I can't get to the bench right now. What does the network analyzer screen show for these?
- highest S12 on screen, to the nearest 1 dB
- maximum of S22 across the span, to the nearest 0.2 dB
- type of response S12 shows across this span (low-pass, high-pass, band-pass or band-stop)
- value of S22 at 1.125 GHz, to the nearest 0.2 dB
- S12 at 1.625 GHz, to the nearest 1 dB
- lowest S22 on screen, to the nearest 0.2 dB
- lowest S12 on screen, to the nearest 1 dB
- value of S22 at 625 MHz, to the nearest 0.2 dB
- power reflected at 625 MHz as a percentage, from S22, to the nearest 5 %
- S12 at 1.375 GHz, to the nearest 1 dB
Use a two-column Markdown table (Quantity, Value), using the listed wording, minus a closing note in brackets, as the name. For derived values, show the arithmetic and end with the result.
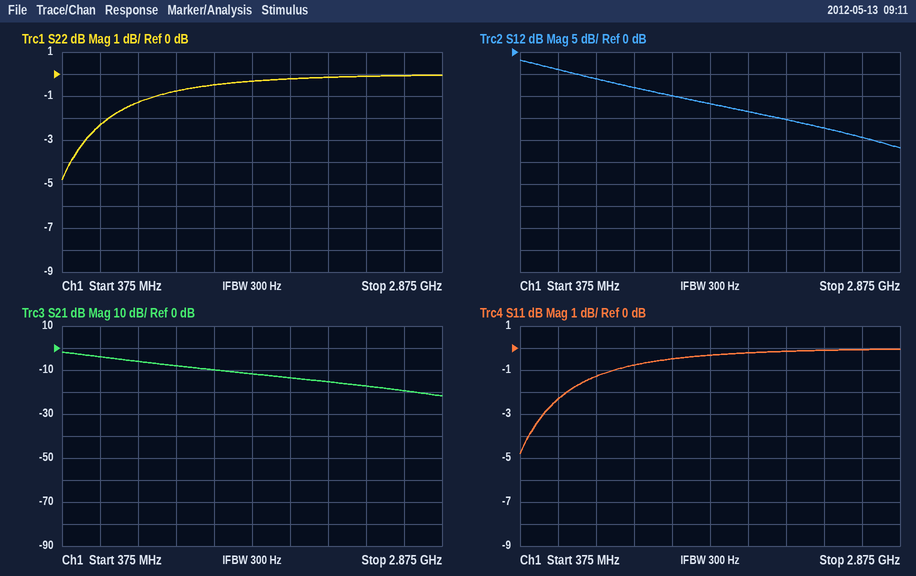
| Quantity | Value |
|---|---|
| highest S12 on screen, to the nearest 1 dB | -2 dB |
| maximum of S22 across the span, to the nearest 0.2 dB | 0.0 dB |
| type of response S12 shows across this span | low-pass |
| value of S22 at 1.125 GHz, to the nearest 0.2 dB | -0.8 dB |
| S12 at 1.625 GHz, to the nearest 1 dB | -12 dB |
| lowest S22 on screen, to the nearest 0.2 dB | -4.8 dB |
| lowest S12 on screen, to the nearest 1 dB | -22 dB |
| value of S22 at 625 MHz, to the nearest 0.2 dB | -2.4 dB |
| power reflected at 625 MHz as a percentage, from S22, to the nearest 5 % | 10^(-2.4/10) ≈ 57.5 %, so 60 % to the nearest 5 % |
| S12 at 1.375 GHz, to the nearest 1 dB | -10 dB |
